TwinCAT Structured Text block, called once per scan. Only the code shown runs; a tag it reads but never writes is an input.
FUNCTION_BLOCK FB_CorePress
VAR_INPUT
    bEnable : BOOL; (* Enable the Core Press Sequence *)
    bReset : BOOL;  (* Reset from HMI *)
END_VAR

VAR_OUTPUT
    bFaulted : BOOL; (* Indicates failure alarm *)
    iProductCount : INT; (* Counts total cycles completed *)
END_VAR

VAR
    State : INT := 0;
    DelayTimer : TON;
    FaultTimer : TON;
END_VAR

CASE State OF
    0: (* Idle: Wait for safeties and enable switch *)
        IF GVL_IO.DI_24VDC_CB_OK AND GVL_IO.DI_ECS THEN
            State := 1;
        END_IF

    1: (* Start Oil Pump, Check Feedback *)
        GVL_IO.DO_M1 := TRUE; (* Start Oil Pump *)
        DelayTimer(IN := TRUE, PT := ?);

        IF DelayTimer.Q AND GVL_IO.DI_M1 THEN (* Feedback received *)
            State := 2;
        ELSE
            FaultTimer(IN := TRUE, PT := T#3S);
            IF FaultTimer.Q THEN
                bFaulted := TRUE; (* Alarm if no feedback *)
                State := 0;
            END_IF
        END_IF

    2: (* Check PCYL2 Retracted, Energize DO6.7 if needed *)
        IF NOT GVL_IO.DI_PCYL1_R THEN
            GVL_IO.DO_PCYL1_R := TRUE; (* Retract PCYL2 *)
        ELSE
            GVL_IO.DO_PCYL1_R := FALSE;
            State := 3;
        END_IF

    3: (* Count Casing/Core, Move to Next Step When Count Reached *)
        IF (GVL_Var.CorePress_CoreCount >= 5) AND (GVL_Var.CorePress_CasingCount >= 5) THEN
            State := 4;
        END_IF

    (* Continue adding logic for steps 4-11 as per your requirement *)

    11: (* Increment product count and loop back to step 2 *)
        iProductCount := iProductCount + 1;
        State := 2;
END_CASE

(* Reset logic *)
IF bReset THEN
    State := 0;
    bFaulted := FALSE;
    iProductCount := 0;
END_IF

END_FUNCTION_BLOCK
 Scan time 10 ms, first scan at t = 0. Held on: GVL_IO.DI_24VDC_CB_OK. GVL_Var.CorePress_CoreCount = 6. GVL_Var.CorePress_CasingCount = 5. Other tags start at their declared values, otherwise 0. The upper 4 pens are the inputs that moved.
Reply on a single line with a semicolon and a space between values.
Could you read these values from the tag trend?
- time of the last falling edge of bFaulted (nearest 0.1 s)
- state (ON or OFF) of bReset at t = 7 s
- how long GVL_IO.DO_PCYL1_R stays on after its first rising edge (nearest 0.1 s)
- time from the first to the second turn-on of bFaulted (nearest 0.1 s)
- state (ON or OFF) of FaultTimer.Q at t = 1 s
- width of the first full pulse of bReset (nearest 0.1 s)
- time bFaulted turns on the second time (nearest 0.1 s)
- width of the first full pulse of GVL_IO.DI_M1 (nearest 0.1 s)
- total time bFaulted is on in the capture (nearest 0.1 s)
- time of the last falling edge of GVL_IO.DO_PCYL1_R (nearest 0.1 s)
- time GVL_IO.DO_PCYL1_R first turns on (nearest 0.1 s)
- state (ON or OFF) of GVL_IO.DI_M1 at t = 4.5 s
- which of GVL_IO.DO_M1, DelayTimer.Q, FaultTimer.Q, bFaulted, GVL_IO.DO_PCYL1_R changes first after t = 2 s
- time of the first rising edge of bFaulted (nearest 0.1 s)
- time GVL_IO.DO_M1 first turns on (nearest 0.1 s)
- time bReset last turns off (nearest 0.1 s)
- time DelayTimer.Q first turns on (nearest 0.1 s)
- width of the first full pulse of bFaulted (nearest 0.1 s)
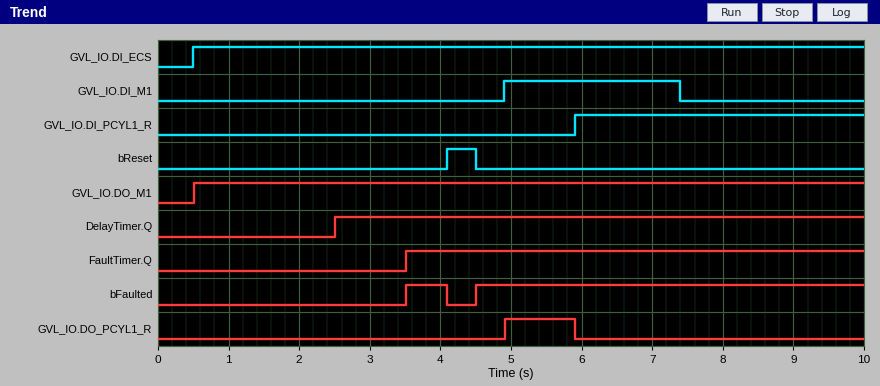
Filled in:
4.1 s; OFF; 1.0 s; 1.0 s; OFF; 0.4 s; 4.5 s; 2.5 s; 6.1 s; 5.9 s; 4.9 s; OFF; DelayTimer.Q; 3.5 s; 0.5 s; 4.5 s; 2.5 s; 0.6 s
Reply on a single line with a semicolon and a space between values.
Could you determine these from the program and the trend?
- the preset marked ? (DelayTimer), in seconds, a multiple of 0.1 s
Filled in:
2.0 s
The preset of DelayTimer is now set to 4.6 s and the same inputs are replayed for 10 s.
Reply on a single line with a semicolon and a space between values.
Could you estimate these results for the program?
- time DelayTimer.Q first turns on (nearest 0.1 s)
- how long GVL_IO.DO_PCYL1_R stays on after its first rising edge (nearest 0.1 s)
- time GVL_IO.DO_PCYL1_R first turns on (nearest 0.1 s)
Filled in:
5.1 s; 0.8 s; 5.1 s
